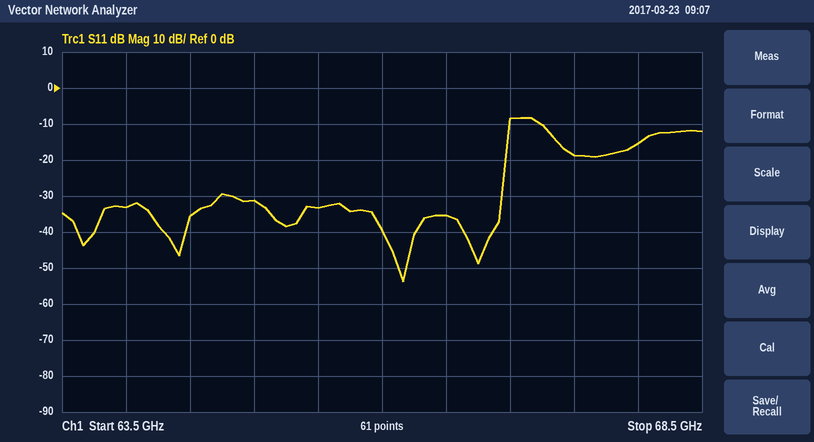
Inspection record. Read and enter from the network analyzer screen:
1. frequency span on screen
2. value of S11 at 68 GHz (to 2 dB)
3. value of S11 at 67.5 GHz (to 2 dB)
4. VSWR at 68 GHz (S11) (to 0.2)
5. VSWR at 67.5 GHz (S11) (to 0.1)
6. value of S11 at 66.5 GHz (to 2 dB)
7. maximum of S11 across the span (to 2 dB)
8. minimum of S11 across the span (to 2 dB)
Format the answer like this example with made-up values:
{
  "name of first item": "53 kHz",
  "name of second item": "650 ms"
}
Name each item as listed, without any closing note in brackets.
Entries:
{
  "frequency span on screen": "5 GHz",
  "value of S11 at 68 GHz": "-16 dB",
  "value of S11 at 67.5 GHz": "-18 dB",
  "VSWR at 68 GHz (S11)": "1.4",
  "VSWR at 67.5 GHz (S11)": "1.3",
  "value of S11 at 66.5 GHz": "-36 dB",
  "maximum of S11 across the span": "-8 dB",
  "minimum of S11 across the span": "-54 dB"
}
